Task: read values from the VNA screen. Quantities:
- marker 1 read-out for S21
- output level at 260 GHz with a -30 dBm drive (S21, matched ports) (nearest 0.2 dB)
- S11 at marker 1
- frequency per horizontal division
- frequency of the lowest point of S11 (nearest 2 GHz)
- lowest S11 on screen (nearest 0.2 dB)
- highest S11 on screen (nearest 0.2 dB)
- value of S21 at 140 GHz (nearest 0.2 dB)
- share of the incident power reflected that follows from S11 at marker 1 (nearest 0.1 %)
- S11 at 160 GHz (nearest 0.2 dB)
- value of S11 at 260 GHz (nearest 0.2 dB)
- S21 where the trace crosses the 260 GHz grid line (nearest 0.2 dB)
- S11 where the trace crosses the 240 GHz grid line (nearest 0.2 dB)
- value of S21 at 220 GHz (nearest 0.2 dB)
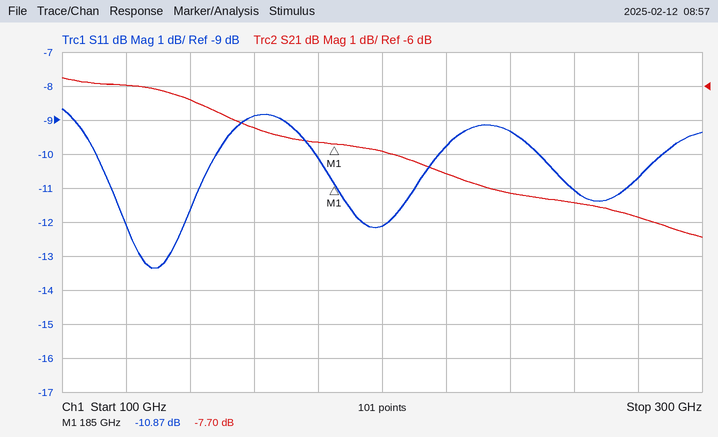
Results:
-7.70 dB
-39.4 dBm
-10.87 dB
20 GHz
128 GHz
-13.4 dB
-8.6 dB
-6.4 dB
8.2 %
-8.8 dB
-11.0 dB
-9.4 dB
-9.4 dB
-8.6 dB
